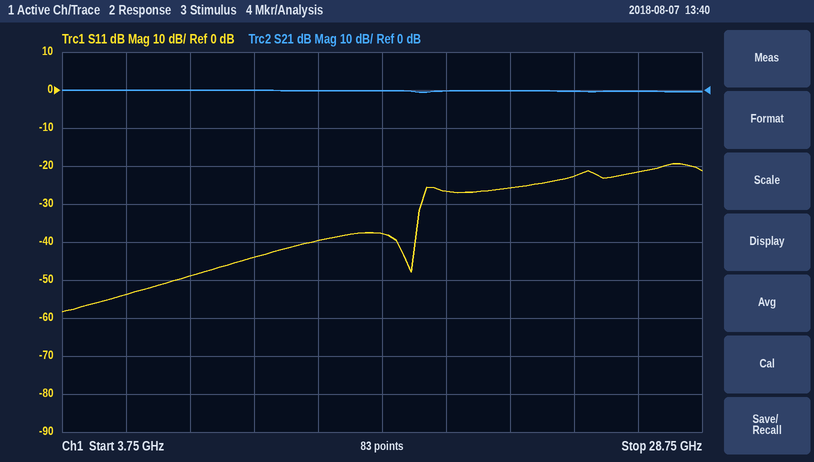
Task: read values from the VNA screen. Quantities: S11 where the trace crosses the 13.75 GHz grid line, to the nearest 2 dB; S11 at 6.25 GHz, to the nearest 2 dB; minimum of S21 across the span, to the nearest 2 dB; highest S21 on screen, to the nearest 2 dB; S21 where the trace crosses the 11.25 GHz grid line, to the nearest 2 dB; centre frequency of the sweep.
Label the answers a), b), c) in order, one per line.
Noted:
a) -40 dB
b) -54 dB
c) 0 dB
d) 0 dB
e) 0 dB
f) 16.25 GHz
